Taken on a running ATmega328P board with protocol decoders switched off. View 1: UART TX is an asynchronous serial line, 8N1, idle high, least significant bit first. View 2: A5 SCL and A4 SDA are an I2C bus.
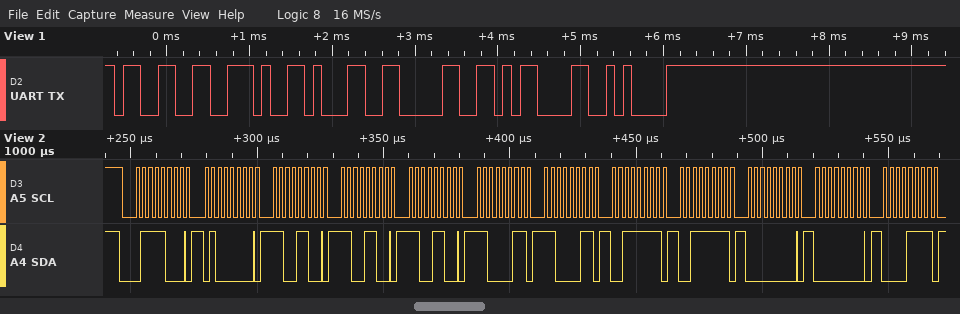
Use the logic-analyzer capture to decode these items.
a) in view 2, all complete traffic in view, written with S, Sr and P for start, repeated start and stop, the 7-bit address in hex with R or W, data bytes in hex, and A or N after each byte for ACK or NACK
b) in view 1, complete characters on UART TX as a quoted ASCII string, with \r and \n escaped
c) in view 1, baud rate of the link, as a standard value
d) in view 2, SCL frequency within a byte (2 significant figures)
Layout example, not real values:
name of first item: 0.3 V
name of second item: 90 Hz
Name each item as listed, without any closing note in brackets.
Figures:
in view 2, all complete traffic in view, written with S, Sr and P for start, repeated start and stop, the 7-bit address in hex with R or W, data bytes in hex, and A or N after each byte for ACK or NACK: S 3CW A 40 A CC A CC A CC A C3 A C3 A 3F A 3F A 00 A 00 A 0F A
in view 1, complete characters on UART TX as a quoted ASCII string, with \r and \n escaped: "3.10\r\n"
in view 1, baud rate of the link, as a standard value: 9600 baud
in view 2, SCL frequency within a byte: 400 kHz
